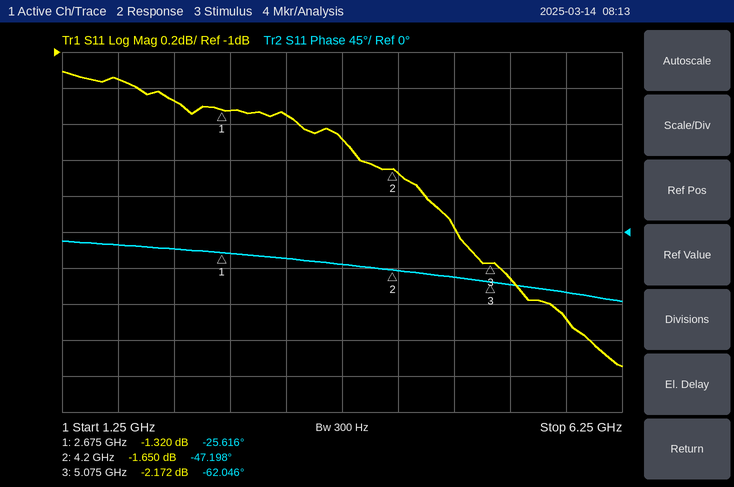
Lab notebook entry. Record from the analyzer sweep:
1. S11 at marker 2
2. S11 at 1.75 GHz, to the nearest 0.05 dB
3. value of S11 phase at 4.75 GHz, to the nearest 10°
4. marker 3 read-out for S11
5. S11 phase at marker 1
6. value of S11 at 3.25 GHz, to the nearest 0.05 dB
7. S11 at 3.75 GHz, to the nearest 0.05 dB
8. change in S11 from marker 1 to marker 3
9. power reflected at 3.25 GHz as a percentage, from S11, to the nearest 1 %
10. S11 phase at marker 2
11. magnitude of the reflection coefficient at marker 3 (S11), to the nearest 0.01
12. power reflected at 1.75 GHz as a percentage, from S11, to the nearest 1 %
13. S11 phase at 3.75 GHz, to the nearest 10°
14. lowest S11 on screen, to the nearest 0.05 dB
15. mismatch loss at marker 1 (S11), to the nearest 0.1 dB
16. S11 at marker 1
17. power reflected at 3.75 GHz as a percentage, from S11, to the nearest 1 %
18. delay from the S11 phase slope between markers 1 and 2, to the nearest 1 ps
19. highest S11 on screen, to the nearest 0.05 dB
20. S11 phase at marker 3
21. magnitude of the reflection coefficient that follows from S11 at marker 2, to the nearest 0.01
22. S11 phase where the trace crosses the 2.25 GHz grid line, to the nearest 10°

-1.650 dB
-1.15 dB
-60°
-2.172 dB
-25.616°
-1.35 dB
-1.50 dB
-0.852 dB
73 %
-47.198°
0.78
77 %
-40°
-2.75 dB
5.8 dB
-1.320 dB
71 %
39 ps
-1.10 dB
-62.046°
0.83
-20°
